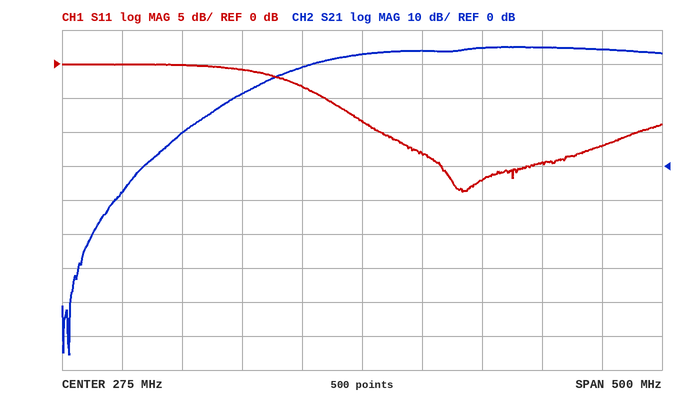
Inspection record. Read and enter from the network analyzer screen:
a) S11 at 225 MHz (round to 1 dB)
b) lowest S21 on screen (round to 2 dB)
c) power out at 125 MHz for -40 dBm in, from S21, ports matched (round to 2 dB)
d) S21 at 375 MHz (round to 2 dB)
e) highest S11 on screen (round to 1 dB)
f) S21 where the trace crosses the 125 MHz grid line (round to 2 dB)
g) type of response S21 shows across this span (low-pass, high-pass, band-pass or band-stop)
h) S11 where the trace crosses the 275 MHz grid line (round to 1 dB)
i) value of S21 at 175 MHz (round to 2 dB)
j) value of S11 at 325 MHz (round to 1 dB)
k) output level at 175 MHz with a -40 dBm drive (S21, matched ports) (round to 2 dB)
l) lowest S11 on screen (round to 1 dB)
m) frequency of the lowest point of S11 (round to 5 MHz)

-3 dB
-56 dB
-30 dBm
34 dB
0 dB
10 dB
high-pass
-8 dB
22 dB
-13 dB
-18 dBm
-19 dB
360 MHz
